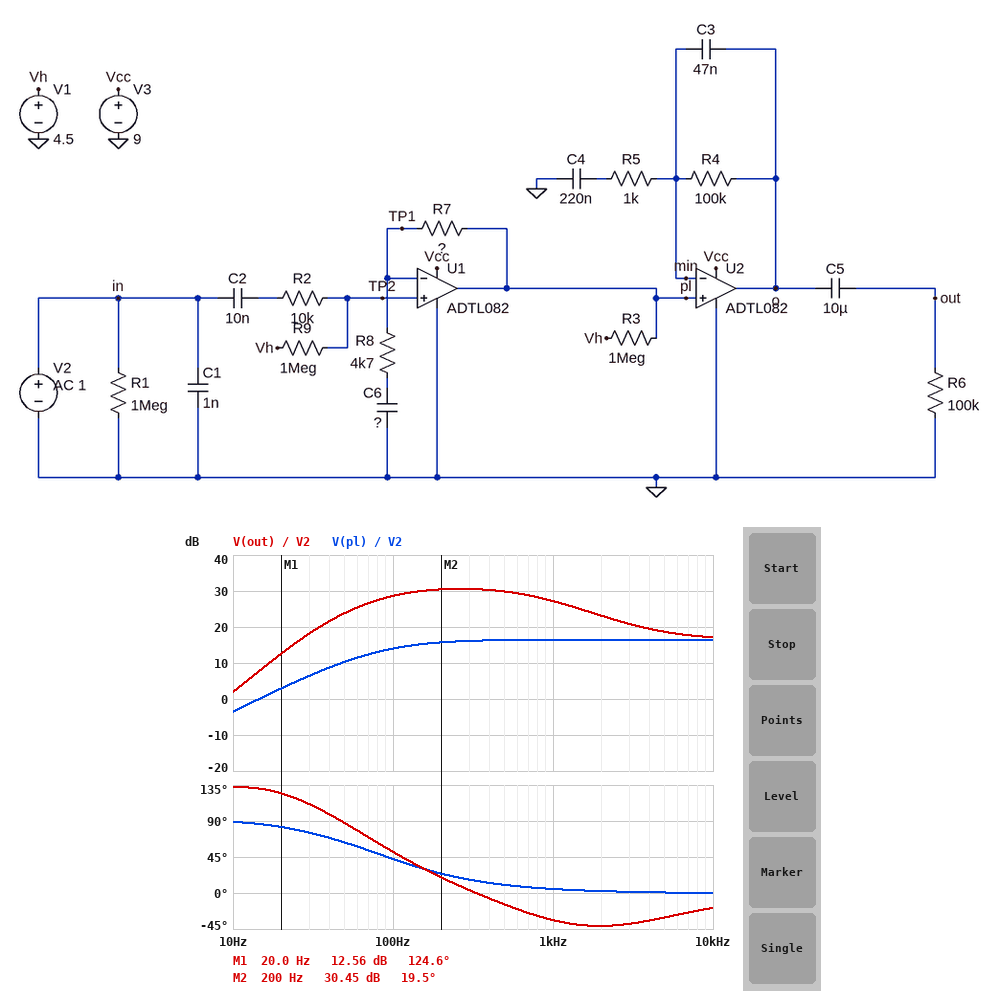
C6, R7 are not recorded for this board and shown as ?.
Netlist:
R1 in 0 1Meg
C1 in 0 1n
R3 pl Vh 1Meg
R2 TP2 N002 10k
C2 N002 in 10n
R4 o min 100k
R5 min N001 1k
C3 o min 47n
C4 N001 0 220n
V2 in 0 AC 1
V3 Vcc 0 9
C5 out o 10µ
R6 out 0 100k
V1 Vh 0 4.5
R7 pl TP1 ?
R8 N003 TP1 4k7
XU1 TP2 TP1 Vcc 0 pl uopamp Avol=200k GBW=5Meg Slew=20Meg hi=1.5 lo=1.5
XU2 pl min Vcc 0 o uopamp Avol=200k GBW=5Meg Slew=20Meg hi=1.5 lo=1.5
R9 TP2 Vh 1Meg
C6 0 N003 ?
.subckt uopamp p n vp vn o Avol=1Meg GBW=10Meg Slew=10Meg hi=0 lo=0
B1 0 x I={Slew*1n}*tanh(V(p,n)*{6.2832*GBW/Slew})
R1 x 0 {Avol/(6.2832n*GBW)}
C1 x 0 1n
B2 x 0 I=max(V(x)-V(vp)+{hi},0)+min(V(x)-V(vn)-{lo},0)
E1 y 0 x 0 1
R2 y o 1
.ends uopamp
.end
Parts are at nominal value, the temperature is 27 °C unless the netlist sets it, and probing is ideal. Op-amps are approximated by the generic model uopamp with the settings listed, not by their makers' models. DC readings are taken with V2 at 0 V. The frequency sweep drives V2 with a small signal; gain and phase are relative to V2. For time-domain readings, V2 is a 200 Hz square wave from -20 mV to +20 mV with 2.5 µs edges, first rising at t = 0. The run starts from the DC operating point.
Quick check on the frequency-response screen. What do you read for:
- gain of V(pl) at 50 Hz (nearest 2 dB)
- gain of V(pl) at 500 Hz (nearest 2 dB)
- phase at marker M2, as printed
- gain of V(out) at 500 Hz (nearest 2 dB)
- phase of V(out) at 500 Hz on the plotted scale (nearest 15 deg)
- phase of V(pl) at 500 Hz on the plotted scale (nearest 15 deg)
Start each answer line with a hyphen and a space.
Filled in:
- 10 dB
- 16 dB
- 19.5 deg
- 30 dB
- -15 deg
- 15 deg
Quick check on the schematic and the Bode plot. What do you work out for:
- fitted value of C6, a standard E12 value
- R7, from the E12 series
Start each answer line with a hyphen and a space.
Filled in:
- 390 nF
- 27 kΩ
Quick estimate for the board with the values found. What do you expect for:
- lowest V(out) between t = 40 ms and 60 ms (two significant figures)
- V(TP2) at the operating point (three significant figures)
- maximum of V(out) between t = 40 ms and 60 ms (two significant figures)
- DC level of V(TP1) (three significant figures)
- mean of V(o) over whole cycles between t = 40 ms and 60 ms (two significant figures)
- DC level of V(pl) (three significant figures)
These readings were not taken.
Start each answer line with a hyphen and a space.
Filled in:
- -950 mV
- 4.50 V
- 950 mV
- 4.50 V
- 4.5 V
- 4.50 V
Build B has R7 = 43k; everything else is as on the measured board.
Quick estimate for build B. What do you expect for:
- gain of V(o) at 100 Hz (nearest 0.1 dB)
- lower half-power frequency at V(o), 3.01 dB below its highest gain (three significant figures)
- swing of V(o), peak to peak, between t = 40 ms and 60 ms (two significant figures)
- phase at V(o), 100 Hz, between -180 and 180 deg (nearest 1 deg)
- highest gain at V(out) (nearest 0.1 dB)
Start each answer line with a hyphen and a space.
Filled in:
- 32.1 dB
- 82.4 Hz
- 2.9 V
- 54 deg
- 34.1 dB
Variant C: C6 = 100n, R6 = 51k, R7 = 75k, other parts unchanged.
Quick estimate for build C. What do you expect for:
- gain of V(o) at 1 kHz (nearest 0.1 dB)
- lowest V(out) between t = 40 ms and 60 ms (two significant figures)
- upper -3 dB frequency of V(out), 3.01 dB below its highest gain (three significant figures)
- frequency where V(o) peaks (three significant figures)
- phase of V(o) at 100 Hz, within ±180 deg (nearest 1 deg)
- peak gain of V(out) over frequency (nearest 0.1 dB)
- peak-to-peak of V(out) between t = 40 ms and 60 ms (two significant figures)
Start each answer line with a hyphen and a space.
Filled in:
- 34.8 dB
- -2.0 V
- 1.34 kHz
- 506 Hz
- 80 deg
- 36.4 dB
- 4.0 V
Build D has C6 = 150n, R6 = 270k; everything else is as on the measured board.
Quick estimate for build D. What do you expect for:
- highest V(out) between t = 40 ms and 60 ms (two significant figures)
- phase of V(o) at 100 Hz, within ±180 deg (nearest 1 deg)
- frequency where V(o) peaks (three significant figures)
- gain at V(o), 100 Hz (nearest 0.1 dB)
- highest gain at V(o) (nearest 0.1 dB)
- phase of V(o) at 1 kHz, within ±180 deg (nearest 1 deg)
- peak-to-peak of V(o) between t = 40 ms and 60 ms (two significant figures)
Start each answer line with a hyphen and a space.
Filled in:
- 880 mV
- 65 deg
- 410 Hz
- 23.6 dB
- 29.3 dB
- -27 deg
- 1.8 V
